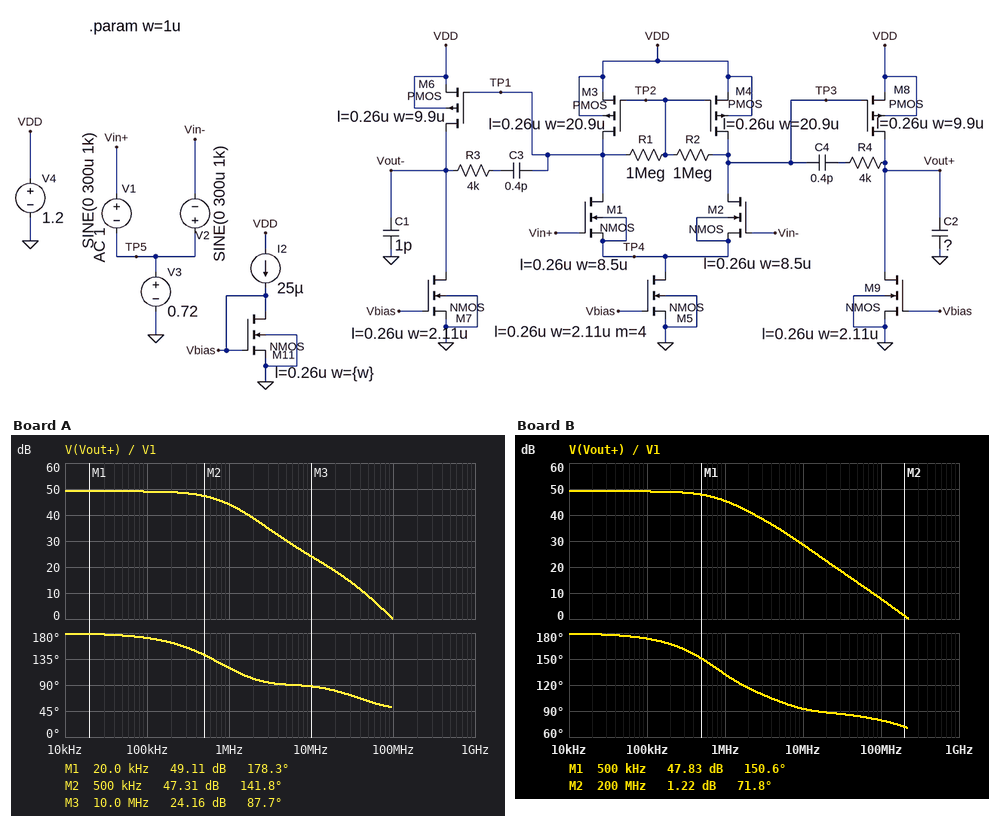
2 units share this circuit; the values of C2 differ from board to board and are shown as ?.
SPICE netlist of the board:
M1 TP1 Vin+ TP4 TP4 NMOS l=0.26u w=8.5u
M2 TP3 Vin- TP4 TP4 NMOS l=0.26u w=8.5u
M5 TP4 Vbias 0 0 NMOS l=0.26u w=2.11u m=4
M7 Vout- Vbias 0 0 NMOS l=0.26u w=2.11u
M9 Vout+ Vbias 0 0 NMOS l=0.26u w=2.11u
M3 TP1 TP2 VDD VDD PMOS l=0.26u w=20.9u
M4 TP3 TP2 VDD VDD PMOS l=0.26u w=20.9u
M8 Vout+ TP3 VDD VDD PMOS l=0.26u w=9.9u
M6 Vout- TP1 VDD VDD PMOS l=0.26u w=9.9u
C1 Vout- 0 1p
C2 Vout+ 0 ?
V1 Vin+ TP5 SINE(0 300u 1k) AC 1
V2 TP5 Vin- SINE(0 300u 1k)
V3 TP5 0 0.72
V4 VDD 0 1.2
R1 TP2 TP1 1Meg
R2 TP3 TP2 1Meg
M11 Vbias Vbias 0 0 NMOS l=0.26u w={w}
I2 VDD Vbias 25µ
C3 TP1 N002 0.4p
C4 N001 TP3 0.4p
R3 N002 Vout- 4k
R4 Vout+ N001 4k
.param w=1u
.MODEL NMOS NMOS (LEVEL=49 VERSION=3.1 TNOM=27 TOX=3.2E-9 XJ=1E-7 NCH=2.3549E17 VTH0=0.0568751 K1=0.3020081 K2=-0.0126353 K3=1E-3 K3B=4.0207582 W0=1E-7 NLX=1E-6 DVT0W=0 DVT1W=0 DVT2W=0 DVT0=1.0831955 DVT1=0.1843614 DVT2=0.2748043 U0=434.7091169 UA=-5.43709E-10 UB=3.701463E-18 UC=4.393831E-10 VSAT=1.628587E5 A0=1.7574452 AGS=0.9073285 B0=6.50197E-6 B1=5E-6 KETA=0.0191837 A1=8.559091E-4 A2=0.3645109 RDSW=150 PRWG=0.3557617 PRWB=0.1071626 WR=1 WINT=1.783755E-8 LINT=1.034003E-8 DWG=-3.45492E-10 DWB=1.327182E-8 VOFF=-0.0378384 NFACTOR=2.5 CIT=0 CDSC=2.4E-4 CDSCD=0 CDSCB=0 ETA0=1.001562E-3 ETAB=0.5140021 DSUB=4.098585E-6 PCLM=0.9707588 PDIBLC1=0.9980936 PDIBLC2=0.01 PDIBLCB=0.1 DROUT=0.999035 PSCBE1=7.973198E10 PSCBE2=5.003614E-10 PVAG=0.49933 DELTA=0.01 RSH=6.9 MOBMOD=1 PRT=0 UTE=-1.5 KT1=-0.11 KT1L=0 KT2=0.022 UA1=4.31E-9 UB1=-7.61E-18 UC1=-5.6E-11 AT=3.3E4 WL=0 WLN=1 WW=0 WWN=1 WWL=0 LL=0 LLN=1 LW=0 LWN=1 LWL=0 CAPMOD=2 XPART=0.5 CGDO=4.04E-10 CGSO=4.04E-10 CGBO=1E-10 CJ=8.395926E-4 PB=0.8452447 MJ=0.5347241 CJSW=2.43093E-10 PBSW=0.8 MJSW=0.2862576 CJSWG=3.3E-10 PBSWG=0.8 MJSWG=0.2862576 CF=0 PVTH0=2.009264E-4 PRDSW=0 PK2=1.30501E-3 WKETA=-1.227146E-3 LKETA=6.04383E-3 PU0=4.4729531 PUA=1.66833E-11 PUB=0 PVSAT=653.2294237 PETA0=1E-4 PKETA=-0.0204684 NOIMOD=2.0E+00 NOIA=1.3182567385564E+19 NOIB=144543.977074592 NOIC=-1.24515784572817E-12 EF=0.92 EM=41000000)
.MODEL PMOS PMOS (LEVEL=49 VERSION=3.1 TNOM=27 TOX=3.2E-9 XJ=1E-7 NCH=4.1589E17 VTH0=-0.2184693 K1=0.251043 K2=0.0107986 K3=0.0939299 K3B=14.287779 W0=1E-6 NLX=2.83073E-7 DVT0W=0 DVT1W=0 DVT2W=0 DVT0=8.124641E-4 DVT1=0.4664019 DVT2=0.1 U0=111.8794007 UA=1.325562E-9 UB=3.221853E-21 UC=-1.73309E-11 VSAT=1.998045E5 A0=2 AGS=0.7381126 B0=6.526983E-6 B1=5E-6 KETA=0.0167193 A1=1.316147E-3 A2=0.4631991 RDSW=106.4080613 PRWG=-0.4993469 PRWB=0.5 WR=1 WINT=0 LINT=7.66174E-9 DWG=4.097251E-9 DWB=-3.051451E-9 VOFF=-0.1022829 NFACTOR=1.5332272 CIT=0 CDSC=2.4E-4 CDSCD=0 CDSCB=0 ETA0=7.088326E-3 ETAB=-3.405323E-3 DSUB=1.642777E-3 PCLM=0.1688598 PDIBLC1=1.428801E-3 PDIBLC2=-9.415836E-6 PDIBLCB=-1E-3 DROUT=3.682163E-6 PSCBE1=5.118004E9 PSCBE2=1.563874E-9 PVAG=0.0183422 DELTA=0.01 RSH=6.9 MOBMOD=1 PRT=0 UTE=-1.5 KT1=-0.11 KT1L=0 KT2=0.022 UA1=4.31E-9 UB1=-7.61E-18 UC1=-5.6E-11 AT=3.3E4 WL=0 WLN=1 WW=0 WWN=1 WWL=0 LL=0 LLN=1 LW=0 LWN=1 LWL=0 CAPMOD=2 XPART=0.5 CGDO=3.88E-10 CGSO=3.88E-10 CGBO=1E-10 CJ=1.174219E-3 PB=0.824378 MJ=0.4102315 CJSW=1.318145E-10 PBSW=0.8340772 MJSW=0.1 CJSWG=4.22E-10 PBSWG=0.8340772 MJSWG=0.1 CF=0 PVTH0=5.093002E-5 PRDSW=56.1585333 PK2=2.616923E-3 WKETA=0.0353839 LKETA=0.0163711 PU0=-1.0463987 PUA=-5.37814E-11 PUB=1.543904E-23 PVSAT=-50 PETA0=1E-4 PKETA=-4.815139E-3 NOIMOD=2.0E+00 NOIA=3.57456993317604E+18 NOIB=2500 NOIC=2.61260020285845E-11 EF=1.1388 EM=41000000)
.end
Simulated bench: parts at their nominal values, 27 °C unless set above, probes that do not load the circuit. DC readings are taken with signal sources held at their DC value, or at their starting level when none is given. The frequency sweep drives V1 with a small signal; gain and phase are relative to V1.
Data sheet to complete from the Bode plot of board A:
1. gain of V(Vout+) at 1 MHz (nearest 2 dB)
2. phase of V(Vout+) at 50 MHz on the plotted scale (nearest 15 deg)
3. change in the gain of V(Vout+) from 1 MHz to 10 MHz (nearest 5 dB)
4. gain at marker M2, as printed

44 dB
60 deg
-20 dB
47.31 dB
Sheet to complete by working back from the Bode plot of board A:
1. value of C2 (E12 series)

2.2 pF
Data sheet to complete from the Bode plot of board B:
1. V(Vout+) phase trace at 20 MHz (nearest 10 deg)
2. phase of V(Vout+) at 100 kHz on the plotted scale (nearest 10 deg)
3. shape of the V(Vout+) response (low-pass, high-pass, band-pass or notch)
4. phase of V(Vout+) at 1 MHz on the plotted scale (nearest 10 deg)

90 deg
170 deg
low-pass
130 deg
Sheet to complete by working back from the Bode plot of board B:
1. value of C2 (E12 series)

560 fF
